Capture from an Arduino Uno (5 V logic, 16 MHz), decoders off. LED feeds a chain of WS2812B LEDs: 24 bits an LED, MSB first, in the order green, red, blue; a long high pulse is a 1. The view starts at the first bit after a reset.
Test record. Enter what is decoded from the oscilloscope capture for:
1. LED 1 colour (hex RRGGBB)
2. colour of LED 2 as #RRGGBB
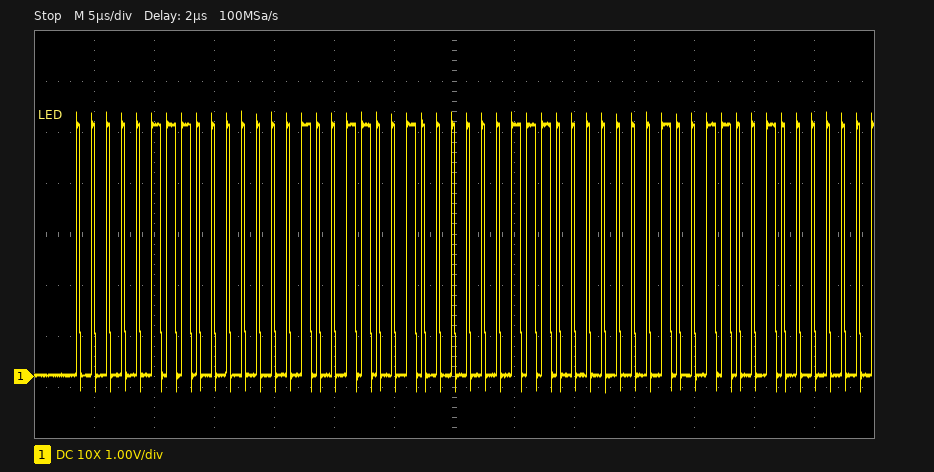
#010732
#010732
